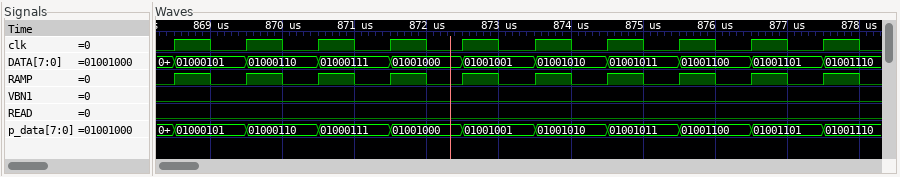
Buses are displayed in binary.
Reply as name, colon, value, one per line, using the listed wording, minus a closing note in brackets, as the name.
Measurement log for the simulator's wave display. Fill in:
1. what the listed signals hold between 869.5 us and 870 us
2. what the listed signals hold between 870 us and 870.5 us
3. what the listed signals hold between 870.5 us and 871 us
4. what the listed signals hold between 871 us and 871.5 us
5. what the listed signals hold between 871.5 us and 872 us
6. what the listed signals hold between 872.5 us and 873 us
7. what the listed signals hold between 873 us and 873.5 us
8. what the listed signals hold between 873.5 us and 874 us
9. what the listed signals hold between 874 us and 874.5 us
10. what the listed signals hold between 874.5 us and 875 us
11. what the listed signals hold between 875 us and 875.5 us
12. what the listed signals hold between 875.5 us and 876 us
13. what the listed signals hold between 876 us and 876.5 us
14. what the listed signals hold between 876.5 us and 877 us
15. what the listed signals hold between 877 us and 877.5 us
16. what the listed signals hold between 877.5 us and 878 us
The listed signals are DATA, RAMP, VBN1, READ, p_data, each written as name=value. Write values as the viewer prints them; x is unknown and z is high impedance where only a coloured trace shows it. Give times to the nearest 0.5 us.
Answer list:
what the listed signals hold between 869.5 us and 870 us: DATA=01000110, RAMP=1, VBN1=0, READ=0, p_data=01000110
what the listed signals hold between 870 us and 870.5 us: DATA=01000110, RAMP=0, VBN1=0, READ=0, p_data=01000110
what the listed signals hold between 870.5 us and 871 us: DATA=01000111, RAMP=1, VBN1=0, READ=0, p_data=01000111
what the listed signals hold between 871 us and 871.5 us: DATA=01000111, RAMP=0, VBN1=0, READ=0, p_data=01000111
what the listed signals hold between 871.5 us and 872 us: DATA=01001000, RAMP=1, VBN1=0, READ=0, p_data=01001000
what the listed signals hold between 872.5 us and 873 us: DATA=01001001, RAMP=1, VBN1=0, READ=0, p_data=01001001
what the listed signals hold between 873 us and 873.5 us: DATA=01001001, RAMP=0, VBN1=0, READ=0, p_data=01001001
what the listed signals hold between 873.5 us and 874 us: DATA=01001010, RAMP=1, VBN1=0, READ=0, p_data=01001010
what the listed signals hold between 874 us and 874.5 us: DATA=01001010, RAMP=0, VBN1=0, READ=0, p_data=01001010
what the listed signals hold between 874.5 us and 875 us: DATA=01001011, RAMP=1, VBN1=0, READ=0, p_data=01001011
what the listed signals hold between 875 us and 875.5 us: DATA=01001011, RAMP=0, VBN1=0, READ=0, p_data=01001011
what the listed signals hold between 875.5 us and 876 us: DATA=01001100, RAMP=1, VBN1=0, READ=0, p_data=01001100
what the listed signals hold between 876 us and 876.5 us: DATA=01001100, RAMP=0, VBN1=0, READ=0, p_data=01001100
what the listed signals hold between 876.5 us and 877 us: DATA=01001101, RAMP=1, VBN1=0, READ=0, p_data=01001101
what the listed signals hold between 877 us and 877.5 us: DATA=01001101, RAMP=0, VBN1=0, READ=0, p_data=01001101
what the listed signals hold between 877.5 us and 878 us: DATA=01001110, RAMP=1, VBN1=0, READ=0, p_data=01001110
